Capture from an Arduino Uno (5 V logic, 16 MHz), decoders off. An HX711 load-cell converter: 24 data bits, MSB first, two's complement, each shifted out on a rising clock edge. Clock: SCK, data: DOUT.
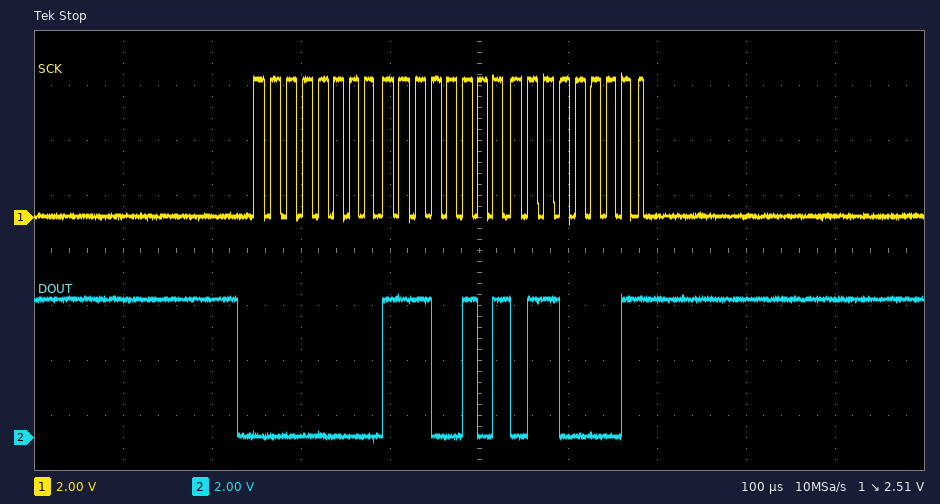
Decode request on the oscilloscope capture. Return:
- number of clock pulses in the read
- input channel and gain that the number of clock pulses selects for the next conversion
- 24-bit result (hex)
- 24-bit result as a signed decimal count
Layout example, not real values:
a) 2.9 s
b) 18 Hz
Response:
a) 25
b) channel A, gain 128
c) 0x00E561
d) 58721
